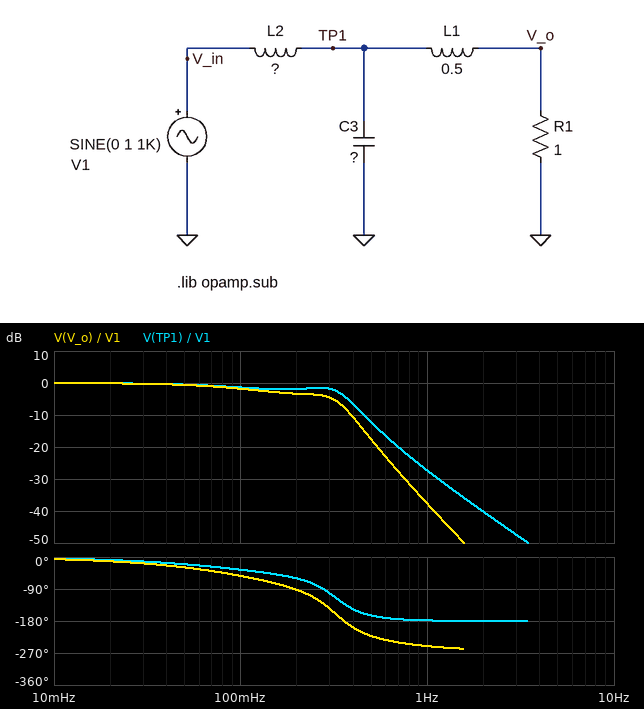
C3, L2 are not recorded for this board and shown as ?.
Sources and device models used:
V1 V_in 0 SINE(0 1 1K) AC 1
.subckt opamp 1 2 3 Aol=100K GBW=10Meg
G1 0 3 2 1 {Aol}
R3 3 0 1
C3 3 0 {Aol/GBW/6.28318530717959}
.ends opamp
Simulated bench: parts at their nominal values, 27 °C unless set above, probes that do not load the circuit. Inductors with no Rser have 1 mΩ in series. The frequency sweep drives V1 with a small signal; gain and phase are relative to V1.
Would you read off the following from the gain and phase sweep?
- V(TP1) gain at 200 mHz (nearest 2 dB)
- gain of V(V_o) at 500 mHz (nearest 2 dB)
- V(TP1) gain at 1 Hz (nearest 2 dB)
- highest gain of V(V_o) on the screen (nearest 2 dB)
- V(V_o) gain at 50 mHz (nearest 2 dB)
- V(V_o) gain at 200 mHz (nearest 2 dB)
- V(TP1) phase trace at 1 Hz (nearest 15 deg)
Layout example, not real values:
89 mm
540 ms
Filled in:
-2 dB
-18 dB
-28 dB
0 dB
0 dB
-4 dB
-180 deg
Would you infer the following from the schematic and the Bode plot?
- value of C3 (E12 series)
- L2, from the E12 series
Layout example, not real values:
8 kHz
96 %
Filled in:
560 mF
1.2 H
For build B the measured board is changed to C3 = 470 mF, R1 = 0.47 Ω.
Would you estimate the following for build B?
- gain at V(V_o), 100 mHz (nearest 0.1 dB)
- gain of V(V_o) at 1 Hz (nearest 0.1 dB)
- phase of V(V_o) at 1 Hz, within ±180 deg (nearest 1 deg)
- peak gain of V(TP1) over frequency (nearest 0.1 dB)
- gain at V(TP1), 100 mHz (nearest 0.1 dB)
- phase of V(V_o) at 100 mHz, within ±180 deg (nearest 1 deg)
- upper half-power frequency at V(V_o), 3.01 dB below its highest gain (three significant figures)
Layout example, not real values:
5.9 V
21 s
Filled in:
-7.1 dB
-42.1 dB
100 deg
1.6 dB
-5.5 dB
-70 deg
46.9 mHz
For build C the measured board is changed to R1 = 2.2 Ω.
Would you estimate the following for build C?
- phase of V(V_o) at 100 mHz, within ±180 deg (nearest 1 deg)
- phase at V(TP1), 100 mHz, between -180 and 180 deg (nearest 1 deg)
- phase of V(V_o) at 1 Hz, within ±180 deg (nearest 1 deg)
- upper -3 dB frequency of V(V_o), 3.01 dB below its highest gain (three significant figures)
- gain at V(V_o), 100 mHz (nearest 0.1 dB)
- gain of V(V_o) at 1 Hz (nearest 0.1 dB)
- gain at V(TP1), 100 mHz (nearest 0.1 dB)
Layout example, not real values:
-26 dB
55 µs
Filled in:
-31 deg
-23 deg
128 deg
254 mHz
1.3 dB
-32.4 dB
1.4 dB
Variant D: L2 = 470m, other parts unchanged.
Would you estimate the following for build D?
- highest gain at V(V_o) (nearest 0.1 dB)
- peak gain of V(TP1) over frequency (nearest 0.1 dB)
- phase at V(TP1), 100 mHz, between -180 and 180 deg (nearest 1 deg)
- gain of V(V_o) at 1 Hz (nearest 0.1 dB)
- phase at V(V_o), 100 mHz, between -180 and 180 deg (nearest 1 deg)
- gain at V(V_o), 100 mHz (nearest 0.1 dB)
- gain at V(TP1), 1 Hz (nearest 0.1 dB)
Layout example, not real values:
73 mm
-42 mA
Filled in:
2.8 dB
6.7 dB
-15 deg
-29.0 dB
-33 deg
-0.6 dB
-18.6 dB
